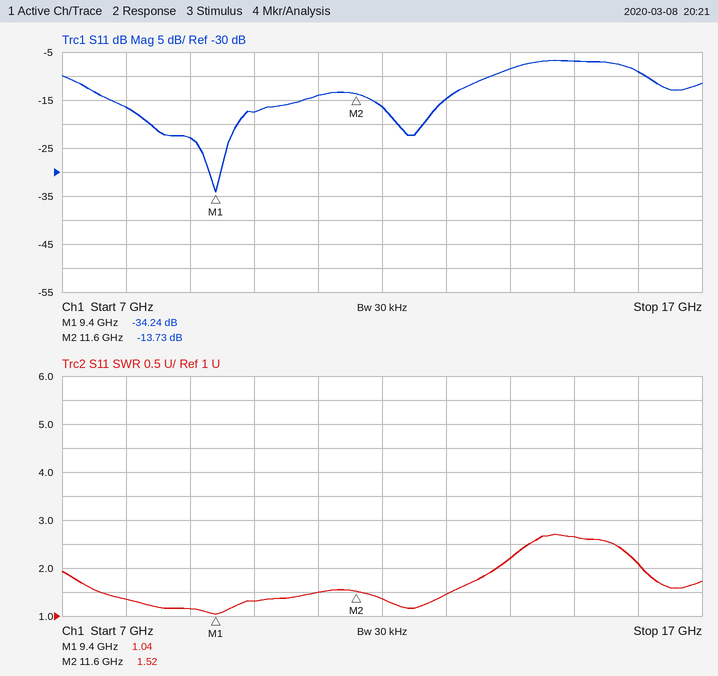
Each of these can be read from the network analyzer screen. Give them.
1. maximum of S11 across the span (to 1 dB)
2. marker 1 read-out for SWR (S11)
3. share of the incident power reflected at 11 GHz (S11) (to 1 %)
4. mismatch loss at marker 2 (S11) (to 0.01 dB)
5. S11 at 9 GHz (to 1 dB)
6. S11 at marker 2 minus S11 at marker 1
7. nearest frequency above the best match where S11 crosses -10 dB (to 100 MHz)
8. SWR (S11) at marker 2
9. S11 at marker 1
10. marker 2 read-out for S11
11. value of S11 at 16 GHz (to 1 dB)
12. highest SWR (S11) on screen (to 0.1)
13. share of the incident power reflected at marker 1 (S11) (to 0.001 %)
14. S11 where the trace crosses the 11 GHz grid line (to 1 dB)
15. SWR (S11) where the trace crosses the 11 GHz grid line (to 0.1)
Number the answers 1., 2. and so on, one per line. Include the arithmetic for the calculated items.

1. -7 dB
2. 1.04
3. 10^(-14/10) ≈ 4 %
4. −10 log10(1 − 10^(-13.73/10)) ≈ 0.19 dB
5. -23 dB
6. -13.73 − (-34.24) = 20.51 dB
7. 13.7 GHz
8. 1.52
9. -34.24 dB
10. -13.73 dB
11. -9 dB
12. 2.7
13. 10^(-34.24/10) ≈ 0.038 %
14. -14 dB
15. 1.5
